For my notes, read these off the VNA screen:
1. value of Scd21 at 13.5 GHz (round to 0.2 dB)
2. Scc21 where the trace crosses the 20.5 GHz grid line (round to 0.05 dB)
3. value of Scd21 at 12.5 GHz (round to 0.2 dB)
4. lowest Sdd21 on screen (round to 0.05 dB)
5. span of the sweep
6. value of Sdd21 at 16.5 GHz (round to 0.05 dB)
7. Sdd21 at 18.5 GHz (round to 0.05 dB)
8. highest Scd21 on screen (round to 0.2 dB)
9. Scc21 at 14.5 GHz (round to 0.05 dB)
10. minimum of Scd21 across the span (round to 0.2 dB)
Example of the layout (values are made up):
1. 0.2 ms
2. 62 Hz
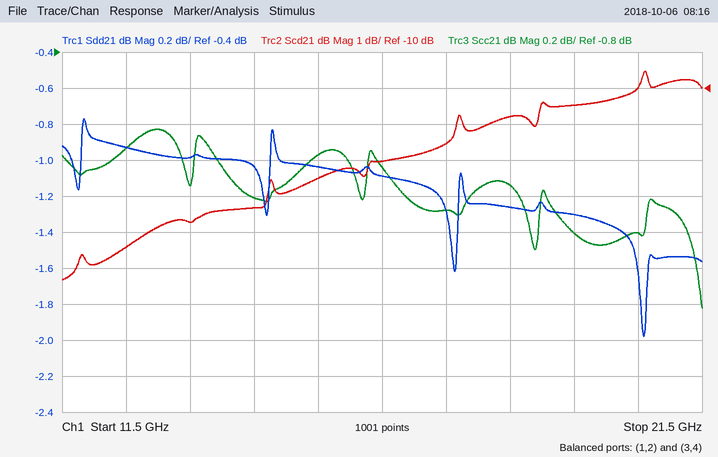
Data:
1. -13.8 dB
2. -1.80 dB
3. -14.4 dB
4. -2.00 dB
5. 10 GHz
6. -1.10 dB
7. -1.25 dB
8. -9.6 dB
9. -1.60 dB
10. -15.4 dB
